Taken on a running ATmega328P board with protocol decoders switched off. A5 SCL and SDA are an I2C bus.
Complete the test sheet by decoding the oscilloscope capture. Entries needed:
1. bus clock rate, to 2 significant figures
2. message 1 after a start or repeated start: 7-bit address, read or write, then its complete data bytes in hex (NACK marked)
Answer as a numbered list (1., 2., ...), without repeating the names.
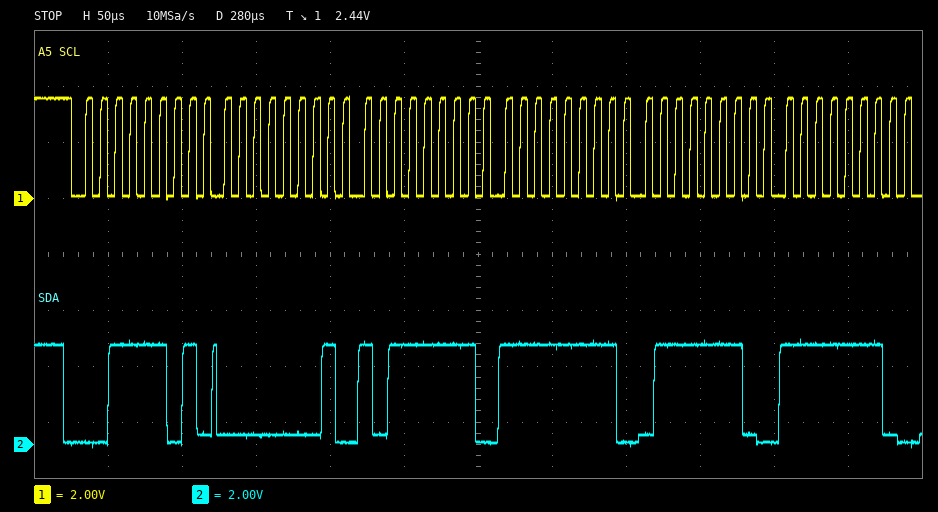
1. 100 kHz
2. 0x1E read: 01 BF FF 7E FE
